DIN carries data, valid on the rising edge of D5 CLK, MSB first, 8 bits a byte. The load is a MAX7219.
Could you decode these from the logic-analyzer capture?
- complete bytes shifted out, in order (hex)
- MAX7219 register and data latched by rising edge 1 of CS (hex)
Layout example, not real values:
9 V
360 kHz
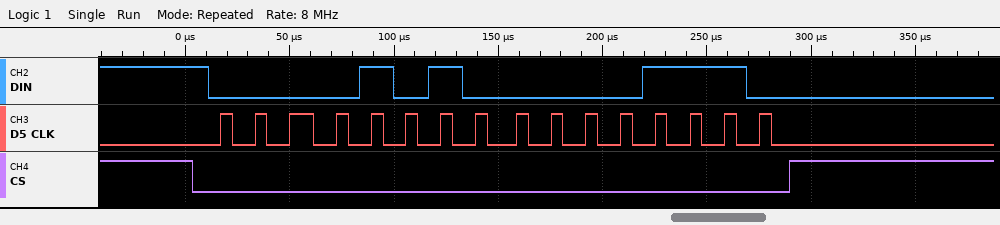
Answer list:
0A 0E
register 0xA, data 0x0E
